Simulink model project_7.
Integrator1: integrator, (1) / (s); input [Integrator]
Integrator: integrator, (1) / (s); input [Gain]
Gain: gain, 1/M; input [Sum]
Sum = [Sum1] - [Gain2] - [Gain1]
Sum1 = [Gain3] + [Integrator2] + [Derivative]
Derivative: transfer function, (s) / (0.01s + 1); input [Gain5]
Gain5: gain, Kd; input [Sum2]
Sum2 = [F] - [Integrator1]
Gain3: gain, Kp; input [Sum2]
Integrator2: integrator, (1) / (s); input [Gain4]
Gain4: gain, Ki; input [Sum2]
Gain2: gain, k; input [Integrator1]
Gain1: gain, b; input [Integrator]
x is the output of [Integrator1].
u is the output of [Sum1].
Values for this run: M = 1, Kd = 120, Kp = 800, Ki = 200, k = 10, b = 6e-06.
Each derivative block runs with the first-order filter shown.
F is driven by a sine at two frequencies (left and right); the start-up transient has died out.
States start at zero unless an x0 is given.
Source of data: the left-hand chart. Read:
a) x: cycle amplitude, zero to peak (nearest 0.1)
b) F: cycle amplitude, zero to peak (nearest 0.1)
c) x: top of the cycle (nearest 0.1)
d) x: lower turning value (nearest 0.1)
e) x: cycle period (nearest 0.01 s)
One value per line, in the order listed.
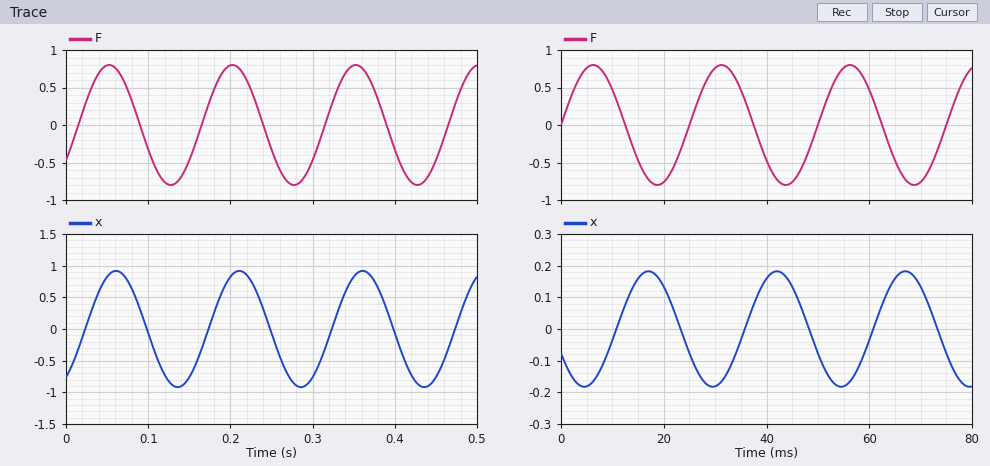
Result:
0.9
0.8
0.9
-0.9
0.15 s
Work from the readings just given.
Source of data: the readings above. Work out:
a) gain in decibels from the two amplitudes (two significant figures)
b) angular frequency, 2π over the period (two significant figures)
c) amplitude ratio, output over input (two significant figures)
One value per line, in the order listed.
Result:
1.0 dB
42 rad/s
1.1
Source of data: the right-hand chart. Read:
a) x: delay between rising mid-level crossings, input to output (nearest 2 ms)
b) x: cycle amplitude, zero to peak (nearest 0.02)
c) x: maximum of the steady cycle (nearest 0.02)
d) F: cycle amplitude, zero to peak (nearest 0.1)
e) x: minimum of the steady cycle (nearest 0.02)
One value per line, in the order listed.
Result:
10 ms
0.18
0.18
0.8
-0.18
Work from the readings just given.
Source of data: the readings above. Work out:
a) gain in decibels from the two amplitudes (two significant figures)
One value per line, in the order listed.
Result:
-13 dB
